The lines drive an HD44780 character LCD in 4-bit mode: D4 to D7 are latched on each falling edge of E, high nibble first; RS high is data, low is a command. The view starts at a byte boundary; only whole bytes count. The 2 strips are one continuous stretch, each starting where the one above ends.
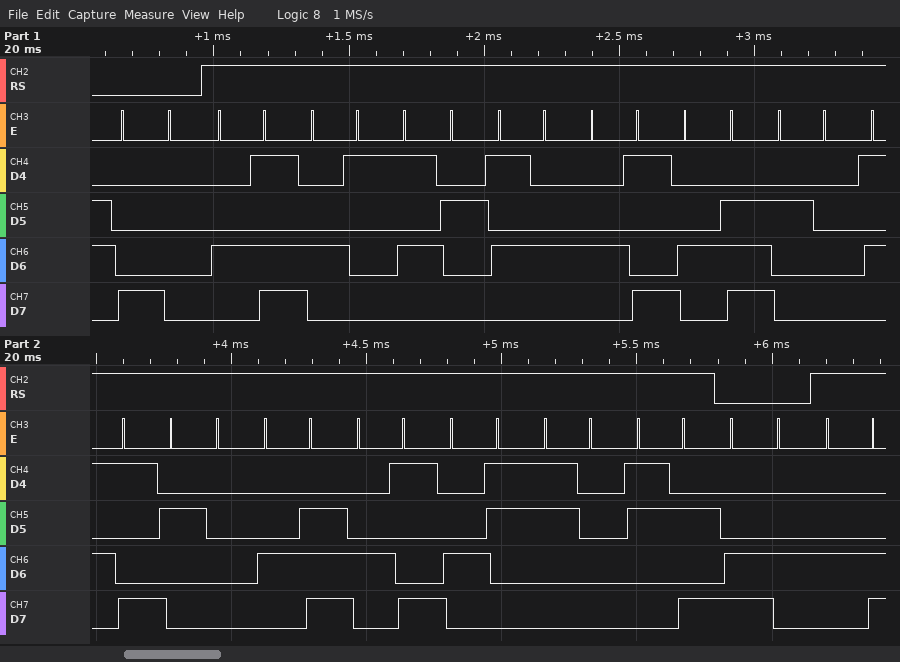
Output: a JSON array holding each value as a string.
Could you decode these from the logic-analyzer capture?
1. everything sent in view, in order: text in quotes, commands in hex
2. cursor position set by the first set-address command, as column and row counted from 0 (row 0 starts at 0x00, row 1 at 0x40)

["0x80 \"MARTIN Y NIC0:\" 0xC4 \"L\"", "column 0, row 0"]
